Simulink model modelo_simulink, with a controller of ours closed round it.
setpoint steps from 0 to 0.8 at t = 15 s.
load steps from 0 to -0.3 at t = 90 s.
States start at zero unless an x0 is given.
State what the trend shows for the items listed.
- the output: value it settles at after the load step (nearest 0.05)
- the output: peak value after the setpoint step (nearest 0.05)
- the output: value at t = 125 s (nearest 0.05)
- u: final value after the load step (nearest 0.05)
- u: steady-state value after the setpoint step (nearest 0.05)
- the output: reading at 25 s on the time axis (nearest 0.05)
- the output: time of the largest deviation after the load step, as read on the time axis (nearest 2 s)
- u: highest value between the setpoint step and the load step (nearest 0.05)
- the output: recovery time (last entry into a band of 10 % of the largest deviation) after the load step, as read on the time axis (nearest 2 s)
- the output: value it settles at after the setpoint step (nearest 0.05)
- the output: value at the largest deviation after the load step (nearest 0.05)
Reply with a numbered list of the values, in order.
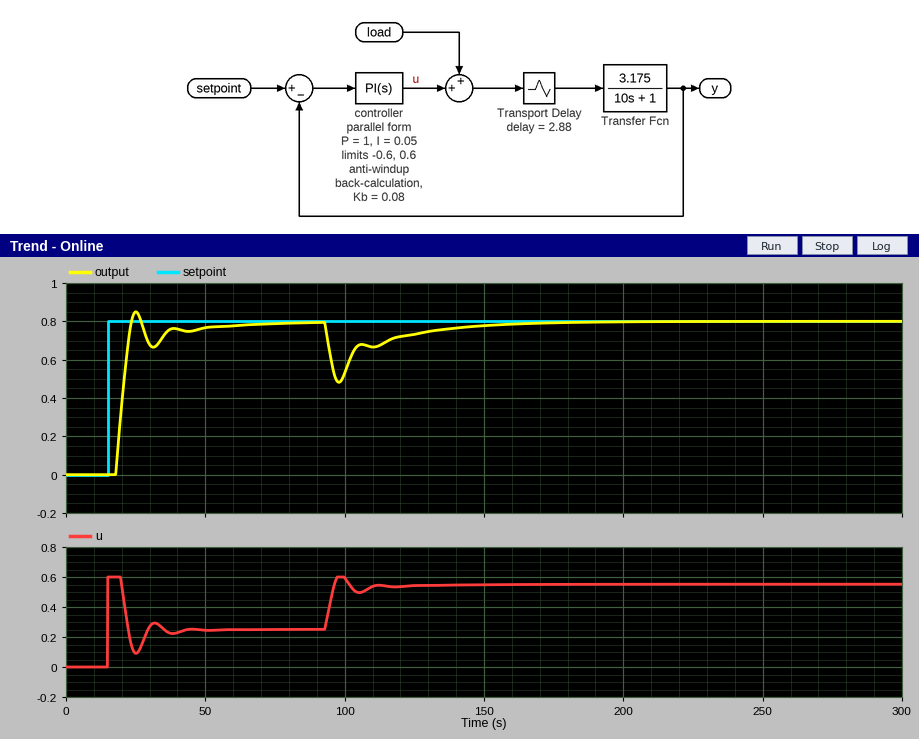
1. 0.80
2. 0.85
3. 0.75
4. 0.55
5. 0.25
6. 0.85
7. 98 s
8. 0.60
9. 142 s
10. 0.80
11. 0.50
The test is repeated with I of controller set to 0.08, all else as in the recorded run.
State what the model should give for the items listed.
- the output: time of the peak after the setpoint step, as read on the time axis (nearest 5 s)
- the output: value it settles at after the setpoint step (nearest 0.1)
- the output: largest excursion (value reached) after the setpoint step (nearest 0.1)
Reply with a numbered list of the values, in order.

1. 25 s
2. 0.8
3. 0.9
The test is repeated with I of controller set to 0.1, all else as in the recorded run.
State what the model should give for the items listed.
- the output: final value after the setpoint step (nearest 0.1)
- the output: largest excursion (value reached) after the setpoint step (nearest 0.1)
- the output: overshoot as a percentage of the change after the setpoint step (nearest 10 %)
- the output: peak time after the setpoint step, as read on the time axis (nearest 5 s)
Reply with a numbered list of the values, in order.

1. 0.8
2. 1.0
3. 20 %
4. 25 s
